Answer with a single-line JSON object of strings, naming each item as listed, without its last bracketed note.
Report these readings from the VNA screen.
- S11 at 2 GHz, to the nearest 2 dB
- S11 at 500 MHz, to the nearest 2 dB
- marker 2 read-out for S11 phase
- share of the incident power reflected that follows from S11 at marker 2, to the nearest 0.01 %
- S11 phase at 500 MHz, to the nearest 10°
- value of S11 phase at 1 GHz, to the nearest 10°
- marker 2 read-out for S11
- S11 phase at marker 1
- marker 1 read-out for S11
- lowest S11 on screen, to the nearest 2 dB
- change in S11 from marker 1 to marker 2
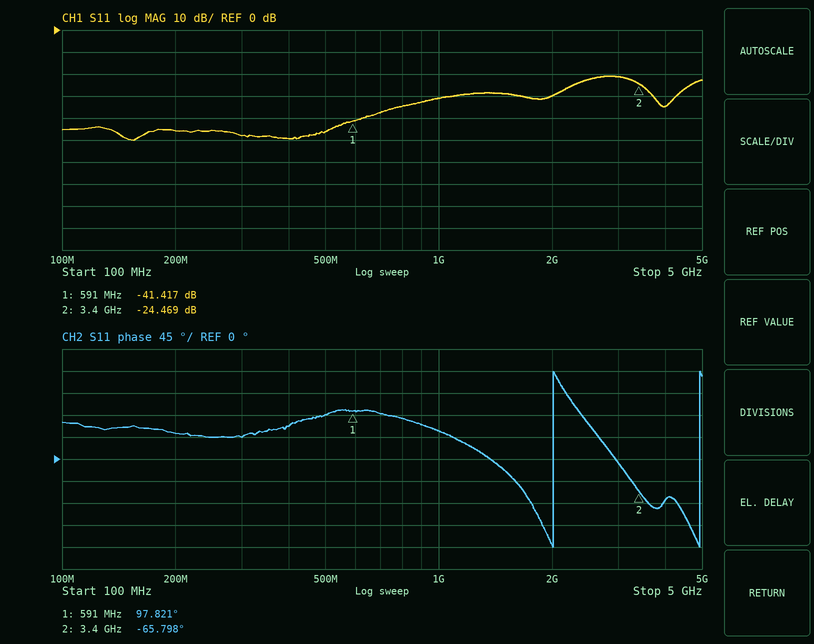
{"S11 at 2 GHz, to the nearest 2 dB": "-30 dB", "S11 at 500 MHz, to the nearest 2 dB": "-46 dB", "marker 2 read-out for S11 phase": "-65.798°", "share of the incident power reflected that follows from S11 at marker 2, to the nearest 0.01 %": "0.36 %", "S11 phase at 500 MHz, to the nearest 10°": "90°", "value of S11 phase at 1 GHz, to the nearest 10°": "60°", "marker 2 read-out for S11": "-24.469 dB", "S11 phase at marker 1": "97.821°", "marker 1 read-out for S11": "-41.417 dB", "lowest S11 on screen, to the nearest 2 dB": "-50 dB", "change in S11 from marker 1 to marker 2": "16.948 dB"}
